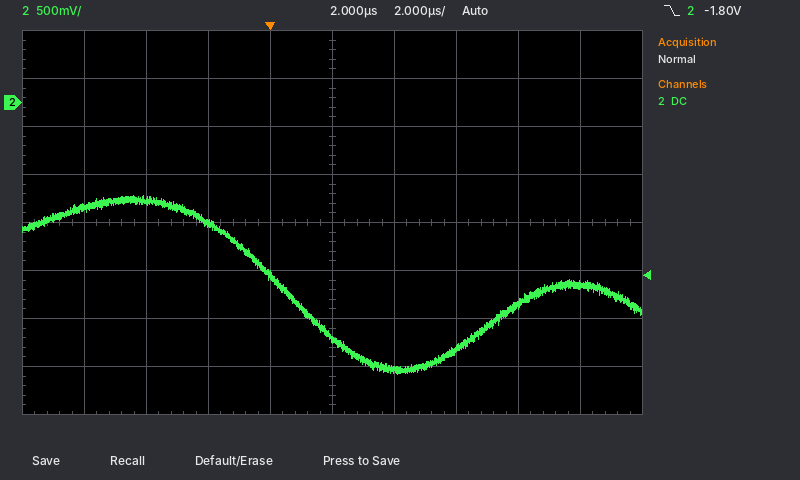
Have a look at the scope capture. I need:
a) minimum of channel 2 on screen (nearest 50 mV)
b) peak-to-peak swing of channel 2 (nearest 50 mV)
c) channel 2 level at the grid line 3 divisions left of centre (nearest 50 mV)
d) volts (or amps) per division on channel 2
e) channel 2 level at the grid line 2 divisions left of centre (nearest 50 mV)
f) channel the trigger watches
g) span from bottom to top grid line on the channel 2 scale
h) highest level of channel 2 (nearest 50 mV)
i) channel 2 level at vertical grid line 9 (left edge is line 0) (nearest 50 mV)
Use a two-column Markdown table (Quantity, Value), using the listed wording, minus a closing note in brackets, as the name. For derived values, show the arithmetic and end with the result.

| Quantity | Value |
|---|---|
| minimum of channel 2 on screen | -2.80 V |
| peak-to-peak swing of channel 2 | -950 mV − (-2.80 V) = 1.85 V |
| channel 2 level at the grid line 3 divisions left of centre | -1.00 V |
| volts (or amps) per division on channel 2 | 500 mV |
| channel 2 level at the grid line 2 divisions left of centre | -1.25 V |
| channel the trigger watches | channel 2 |
| span from bottom to top grid line on the channel 2 scale | 4 V |
| highest level of channel 2 | -950 mV |
| channel 2 level at vertical grid line 9 (left edge is line 0) | -1.90 V |
